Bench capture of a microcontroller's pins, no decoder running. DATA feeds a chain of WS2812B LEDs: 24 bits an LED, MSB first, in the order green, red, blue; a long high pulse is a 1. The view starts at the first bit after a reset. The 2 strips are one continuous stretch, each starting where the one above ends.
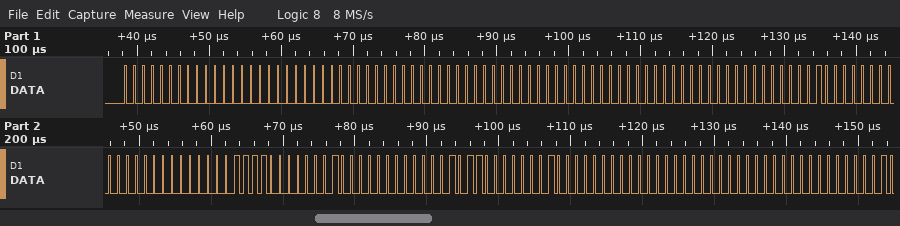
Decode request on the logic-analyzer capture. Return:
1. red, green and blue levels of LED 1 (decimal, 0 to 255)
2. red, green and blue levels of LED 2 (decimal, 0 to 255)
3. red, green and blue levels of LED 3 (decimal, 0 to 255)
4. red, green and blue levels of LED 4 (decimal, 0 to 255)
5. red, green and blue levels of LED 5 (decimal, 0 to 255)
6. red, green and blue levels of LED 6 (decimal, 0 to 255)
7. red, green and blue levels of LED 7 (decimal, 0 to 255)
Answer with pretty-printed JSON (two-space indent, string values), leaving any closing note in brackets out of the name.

{
  "red, green and blue levels of LED 1": "0, 0, 0",
  "red, green and blue levels of LED 2": "0, 0, 0",
  "red, green and blue levels of LED 3": "0, 0, 0",
  "red, green and blue levels of LED 4": "0, 4, 0",
  "red, green and blue levels of LED 5": "1, 15, 0",
  "red, green and blue levels of LED 6": "1, 11, 0",
  "red, green and blue levels of LED 7": "0, 0, 0"
}
